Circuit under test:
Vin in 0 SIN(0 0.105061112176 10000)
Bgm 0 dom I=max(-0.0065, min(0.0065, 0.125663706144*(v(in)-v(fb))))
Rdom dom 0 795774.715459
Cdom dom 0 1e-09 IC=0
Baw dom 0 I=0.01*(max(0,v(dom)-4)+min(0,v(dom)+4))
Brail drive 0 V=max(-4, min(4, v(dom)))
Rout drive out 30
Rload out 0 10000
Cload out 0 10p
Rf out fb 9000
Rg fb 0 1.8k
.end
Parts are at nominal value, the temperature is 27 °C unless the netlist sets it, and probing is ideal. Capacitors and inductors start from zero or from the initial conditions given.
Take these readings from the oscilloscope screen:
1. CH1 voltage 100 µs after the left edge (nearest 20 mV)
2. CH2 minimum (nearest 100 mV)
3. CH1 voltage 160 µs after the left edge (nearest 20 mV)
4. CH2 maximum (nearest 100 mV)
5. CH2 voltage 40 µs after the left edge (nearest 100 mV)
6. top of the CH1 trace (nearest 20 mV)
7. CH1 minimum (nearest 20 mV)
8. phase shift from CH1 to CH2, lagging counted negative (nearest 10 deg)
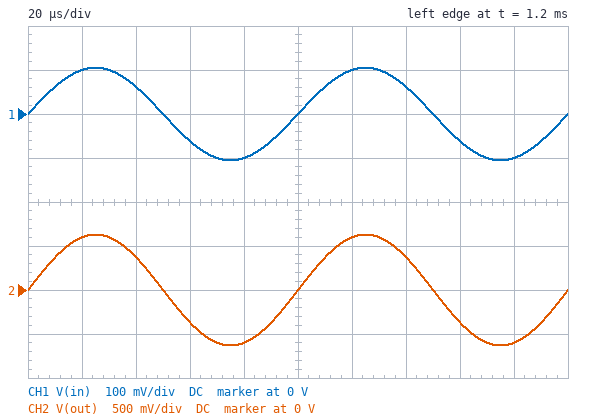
0 V
-600 mV
-60 mV
600 mV
400 mV
100 mV
-100 mV
0 deg
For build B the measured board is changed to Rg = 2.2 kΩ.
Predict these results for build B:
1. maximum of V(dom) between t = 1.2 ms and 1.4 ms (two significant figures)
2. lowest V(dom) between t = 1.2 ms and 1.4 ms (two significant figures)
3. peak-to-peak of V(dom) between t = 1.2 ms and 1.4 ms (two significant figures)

540 mV
-540 mV
1.1 V
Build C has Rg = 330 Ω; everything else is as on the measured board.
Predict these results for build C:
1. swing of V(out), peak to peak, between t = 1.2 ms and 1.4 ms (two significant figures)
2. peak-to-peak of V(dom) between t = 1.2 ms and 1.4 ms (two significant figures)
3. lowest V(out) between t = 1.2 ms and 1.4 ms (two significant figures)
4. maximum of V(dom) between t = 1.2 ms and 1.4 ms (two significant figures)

5.9 V
6.0 V
-3.0 V
3.0 V
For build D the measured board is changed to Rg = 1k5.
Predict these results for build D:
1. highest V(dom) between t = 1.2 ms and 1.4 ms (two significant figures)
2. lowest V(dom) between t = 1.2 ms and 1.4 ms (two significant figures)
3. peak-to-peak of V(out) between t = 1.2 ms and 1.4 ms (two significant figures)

740 mV
-740 mV
1.5 V
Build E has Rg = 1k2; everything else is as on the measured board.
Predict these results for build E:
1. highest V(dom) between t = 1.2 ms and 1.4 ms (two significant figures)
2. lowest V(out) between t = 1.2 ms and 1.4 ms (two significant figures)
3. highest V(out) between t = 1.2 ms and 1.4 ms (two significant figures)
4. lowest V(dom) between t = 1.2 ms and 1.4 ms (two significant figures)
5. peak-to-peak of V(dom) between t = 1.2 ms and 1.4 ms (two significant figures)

900 mV
-890 mV
890 mV
-900 mV
1.8 V
